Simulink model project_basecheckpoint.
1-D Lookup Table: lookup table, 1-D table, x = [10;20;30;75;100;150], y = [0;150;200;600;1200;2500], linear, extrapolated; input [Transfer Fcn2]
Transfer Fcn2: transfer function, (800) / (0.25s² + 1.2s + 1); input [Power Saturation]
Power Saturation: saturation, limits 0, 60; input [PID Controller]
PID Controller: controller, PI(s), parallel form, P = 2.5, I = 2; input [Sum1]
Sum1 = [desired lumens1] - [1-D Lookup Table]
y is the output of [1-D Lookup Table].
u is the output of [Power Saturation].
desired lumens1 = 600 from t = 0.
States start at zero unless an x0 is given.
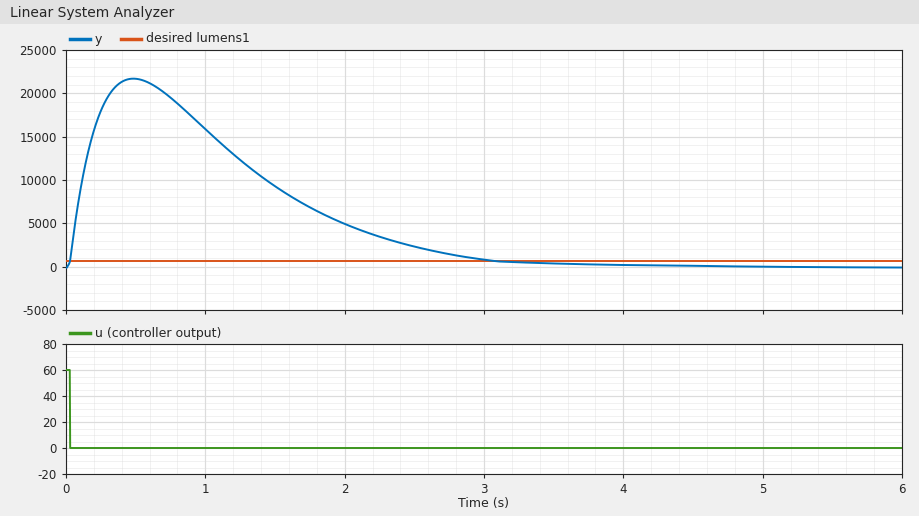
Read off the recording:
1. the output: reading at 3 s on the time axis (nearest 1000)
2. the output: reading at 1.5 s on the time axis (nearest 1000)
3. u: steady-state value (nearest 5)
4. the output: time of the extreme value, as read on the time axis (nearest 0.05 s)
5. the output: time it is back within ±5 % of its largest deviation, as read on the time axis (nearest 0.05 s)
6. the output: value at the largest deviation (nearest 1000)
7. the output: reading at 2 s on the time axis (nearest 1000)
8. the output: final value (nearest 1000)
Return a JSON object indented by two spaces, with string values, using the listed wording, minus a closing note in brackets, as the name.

{
  "the output: reading at 3 s on the time axis": "1000",
  "the output: reading at 1.5 s on the time axis": "9000",
  "u: steady-state value": "0",
  "the output: time of the extreme value, as read on the time axis": "0.50 s",
  "the output: time it is back within ±5 % of its largest deviation, as read on the time axis": "2.95 s",
  "the output: value at the largest deviation": "22000",
  "the output: reading at 2 s on the time axis": "5000",
  "the output: final value": "0"
}
